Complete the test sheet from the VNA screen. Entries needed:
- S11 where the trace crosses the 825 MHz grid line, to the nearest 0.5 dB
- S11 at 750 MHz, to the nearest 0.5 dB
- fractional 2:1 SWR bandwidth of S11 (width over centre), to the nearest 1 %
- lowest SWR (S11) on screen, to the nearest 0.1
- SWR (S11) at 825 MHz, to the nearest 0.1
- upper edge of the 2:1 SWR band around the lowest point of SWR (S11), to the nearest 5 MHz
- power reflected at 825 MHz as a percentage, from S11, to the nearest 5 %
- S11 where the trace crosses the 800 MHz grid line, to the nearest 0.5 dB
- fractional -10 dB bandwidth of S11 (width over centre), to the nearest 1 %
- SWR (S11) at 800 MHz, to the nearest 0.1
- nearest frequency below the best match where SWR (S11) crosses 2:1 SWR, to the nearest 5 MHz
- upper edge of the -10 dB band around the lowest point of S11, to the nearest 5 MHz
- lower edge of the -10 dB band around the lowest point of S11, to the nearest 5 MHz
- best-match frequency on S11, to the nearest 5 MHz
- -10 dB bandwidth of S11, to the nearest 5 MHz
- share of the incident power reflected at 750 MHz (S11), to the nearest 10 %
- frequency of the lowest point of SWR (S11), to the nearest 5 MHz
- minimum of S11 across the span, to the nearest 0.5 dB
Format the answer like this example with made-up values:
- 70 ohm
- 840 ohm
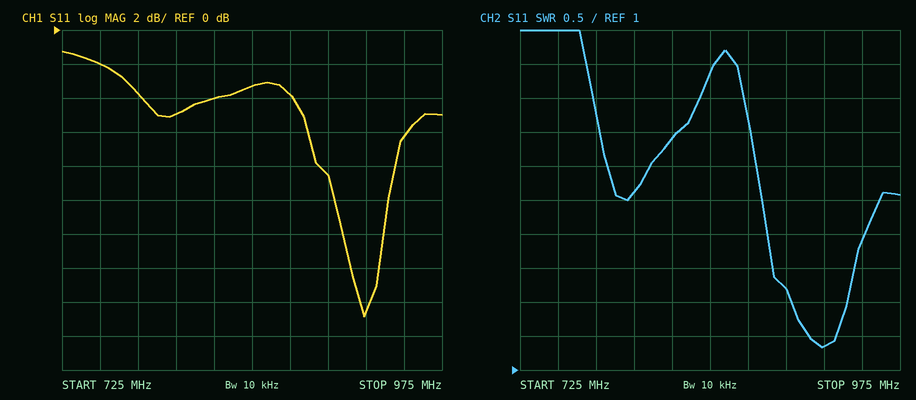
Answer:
- -4.0 dB
- -2.0 dB
- 4 %
- 1.3
- 4.4
- 940 MHz
- 40 %
- -5.0 dB
- 4 %
- 3.6
- 905 MHz
- 940 MHz
- 905 MHz
- 925 MHz
- 35 MHz
- 60 %
- 925 MHz
- -17.0 dB
